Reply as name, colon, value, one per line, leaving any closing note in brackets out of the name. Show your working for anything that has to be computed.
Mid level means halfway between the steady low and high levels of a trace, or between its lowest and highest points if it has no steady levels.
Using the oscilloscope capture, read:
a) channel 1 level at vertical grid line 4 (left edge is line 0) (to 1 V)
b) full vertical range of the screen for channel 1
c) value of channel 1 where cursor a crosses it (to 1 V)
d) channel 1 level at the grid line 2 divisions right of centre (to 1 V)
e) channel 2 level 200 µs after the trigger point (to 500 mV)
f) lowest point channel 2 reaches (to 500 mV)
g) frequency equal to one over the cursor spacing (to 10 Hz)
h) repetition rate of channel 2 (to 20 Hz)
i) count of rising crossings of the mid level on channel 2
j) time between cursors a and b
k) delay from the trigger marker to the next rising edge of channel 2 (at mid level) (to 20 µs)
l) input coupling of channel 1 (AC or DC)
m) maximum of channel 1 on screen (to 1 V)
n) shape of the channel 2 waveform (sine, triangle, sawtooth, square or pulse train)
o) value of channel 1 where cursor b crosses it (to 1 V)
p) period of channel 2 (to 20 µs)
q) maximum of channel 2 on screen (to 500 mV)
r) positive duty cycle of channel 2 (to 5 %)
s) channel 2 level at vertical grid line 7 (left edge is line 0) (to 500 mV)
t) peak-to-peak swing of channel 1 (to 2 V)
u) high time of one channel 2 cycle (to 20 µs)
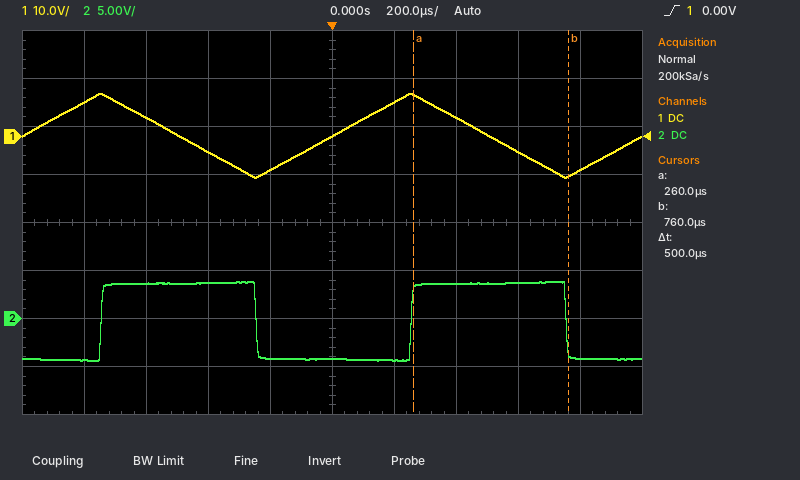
channel 1 level at vertical grid line 4 (left edge is line 0): -7 V
full vertical range of the screen for channel 1: 80 V
value of channel 1 where cursor a crosses it: 9 V
channel 1 level at the grid line 2 divisions right of centre: 4 V
channel 2 level 200 µs after the trigger point: -4.5 V
lowest point channel 2 reaches: -4.5 V
frequency equal to one over the cursor spacing: 1 / 500 µs ≈ 2.00 kHz
repetition rate of channel 2: 1 / 1.00 ms ≈ 1.00 kHz
count of rising crossings of the mid level on channel 2: 2
time between cursors a and b: 500 µs
delay from the trigger marker to the next rising edge of channel 2 (at mid level): 260 µs
input coupling of channel 1: DC
maximum of channel 1 on screen: 9 V
shape of the channel 2 waveform: square
value of channel 1 where cursor b crosses it: -8 V
period of channel 2: 1.00 ms
maximum of channel 2 on screen: 4.0 V
positive duty cycle of channel 2: 500 µs / 1.00 ms ≈ 50 %
channel 2 level at vertical grid line 7 (left edge is line 0): 3.5 V
peak-to-peak swing of channel 1: 18 V
high time of one channel 2 cycle: 500 µs
